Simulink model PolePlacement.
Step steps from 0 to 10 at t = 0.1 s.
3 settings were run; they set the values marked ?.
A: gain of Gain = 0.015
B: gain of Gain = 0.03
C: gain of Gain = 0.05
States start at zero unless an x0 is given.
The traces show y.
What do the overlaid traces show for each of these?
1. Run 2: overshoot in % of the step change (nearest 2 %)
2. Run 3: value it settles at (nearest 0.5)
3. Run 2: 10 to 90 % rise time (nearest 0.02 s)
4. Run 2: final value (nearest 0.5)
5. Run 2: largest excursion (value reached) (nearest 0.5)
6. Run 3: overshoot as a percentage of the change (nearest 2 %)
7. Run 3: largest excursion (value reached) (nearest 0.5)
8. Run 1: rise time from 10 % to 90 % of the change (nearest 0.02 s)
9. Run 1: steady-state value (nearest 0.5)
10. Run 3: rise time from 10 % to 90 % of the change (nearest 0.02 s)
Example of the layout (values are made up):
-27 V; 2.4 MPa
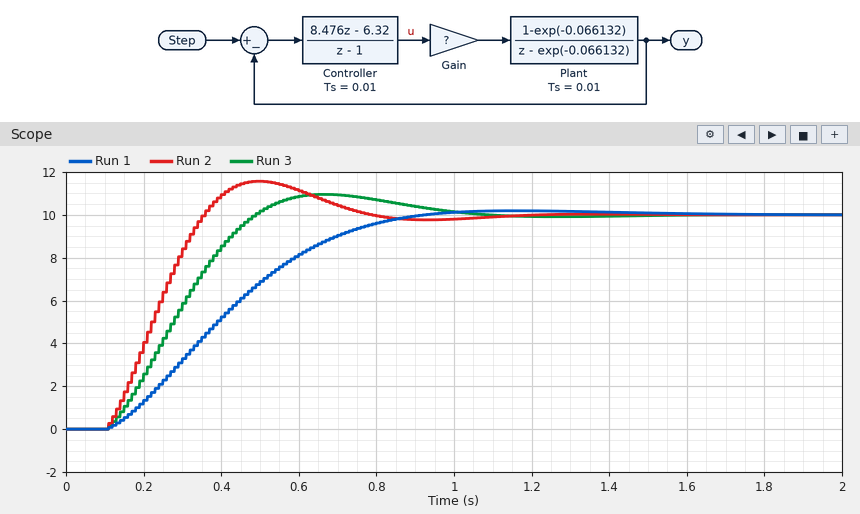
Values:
16 %; 10.0; 0.18 s; 10.0; 11.5; 10 %; 11.0; 0.52 s; 10.0; 0.28 s
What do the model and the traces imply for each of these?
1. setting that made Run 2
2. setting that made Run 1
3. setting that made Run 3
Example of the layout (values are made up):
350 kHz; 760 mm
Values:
C; A; B
